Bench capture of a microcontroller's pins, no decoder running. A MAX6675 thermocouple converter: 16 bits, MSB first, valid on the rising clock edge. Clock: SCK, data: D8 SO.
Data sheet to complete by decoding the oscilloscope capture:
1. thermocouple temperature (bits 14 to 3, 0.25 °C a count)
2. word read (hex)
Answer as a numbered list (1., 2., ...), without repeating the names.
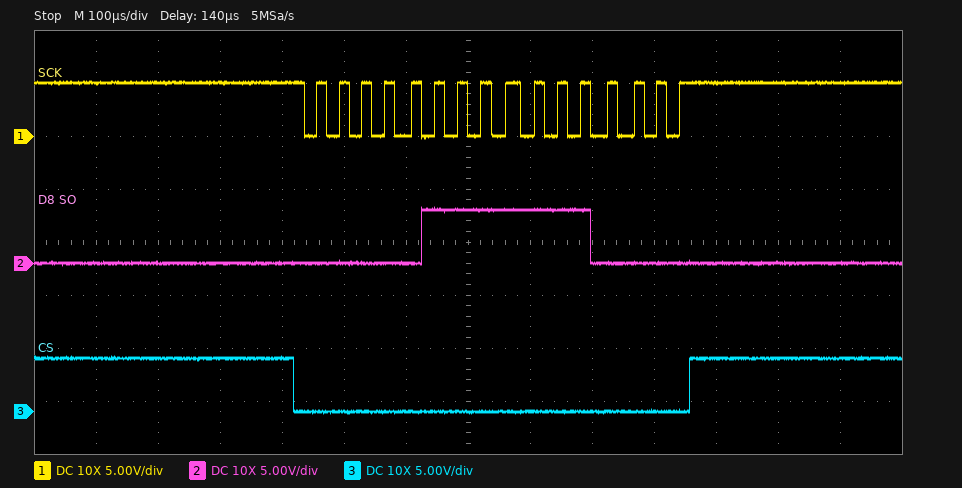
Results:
1. 63.50 °C
2. 0x07F0
